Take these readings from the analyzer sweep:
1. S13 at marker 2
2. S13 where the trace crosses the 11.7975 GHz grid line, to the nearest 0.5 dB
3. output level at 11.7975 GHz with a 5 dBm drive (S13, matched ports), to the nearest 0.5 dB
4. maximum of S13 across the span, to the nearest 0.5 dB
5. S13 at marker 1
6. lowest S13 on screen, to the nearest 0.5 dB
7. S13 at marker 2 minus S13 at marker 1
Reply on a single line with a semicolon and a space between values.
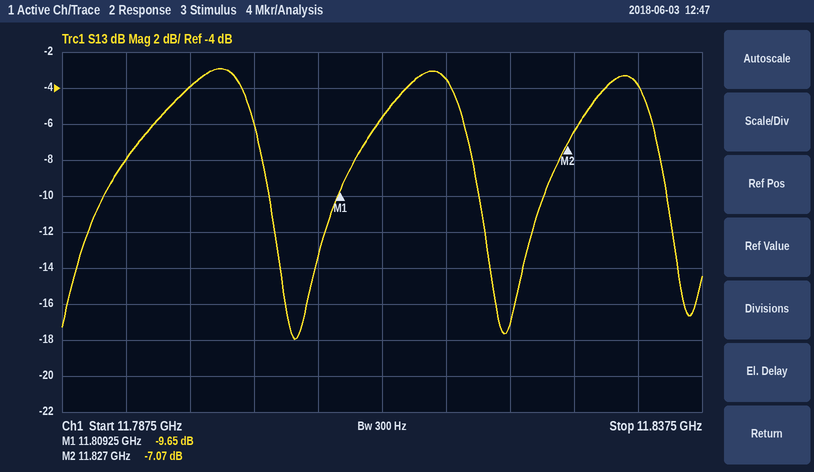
-7.07 dB; -4.0 dB; 1.0 dBm; -3.0 dB; -9.65 dB; -18.0 dB; 2.58 dB
